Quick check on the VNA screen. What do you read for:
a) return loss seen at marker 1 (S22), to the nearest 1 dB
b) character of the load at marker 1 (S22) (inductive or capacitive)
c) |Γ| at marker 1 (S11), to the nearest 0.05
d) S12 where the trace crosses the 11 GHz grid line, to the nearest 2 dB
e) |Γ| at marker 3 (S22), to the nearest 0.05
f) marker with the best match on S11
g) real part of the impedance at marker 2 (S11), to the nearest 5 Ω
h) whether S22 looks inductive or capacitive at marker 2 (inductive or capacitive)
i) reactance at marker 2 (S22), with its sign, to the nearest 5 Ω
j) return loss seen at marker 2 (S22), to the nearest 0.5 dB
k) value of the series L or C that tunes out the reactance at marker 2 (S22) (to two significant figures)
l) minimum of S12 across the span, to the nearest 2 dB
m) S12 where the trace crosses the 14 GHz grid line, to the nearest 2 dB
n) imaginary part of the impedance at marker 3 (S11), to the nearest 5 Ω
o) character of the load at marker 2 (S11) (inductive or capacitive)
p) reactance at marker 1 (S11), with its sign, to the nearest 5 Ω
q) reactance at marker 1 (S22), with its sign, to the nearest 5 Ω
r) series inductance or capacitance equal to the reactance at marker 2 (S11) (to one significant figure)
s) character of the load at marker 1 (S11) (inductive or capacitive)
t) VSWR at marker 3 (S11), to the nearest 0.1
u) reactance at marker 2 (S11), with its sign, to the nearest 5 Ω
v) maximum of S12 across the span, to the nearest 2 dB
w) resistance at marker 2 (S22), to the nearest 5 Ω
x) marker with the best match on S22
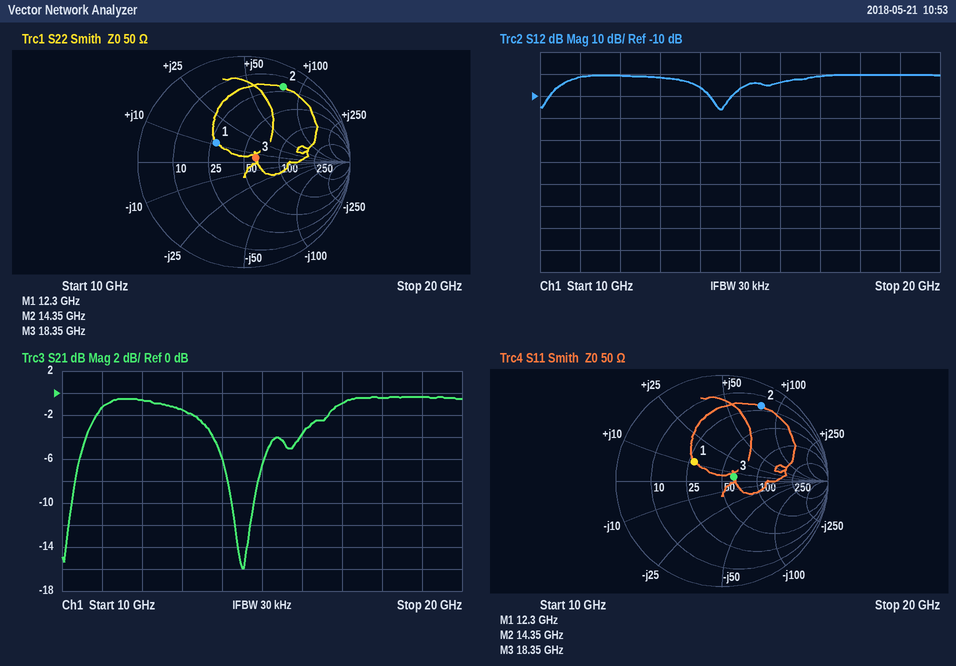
10 dB
inductive
0.30
-2 dB
0.10
marker 3
20 Ω
inductive
+80 Ω
2.0 dB
140 fF
-16 dB
-6 dB
+5 Ω
inductive
+10 Ω
+10 Ω
900 pH
inductive
1.3
+80 Ω
0 dB
20 Ω
marker 3
